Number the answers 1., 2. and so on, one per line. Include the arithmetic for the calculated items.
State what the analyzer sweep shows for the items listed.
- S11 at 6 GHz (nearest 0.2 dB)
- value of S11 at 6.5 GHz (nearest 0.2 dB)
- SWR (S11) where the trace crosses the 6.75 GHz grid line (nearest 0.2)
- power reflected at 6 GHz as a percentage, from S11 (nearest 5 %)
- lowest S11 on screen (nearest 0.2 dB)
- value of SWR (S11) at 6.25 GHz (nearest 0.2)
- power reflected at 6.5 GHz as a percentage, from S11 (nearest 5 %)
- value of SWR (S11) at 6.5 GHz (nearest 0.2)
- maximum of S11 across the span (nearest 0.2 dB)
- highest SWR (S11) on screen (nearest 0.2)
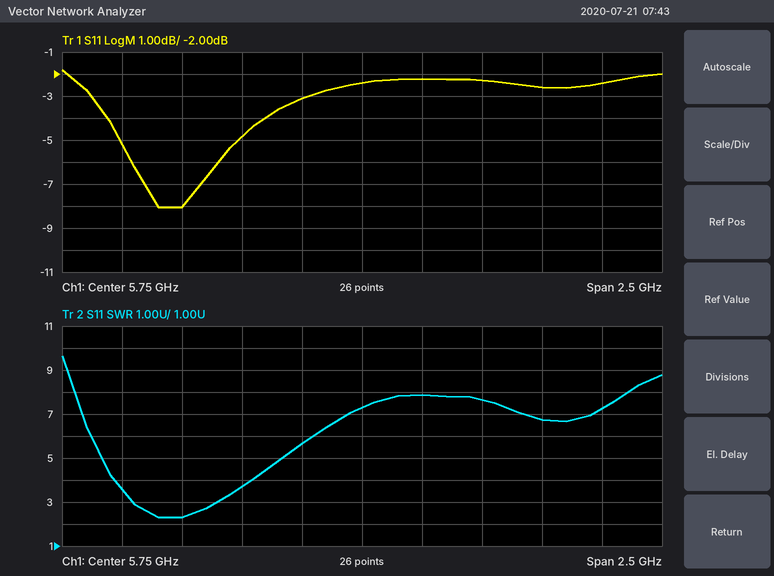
1. -2.2 dB
2. -2.6 dB
3. 7.2
4. 10^(-2.2/10) ≈ 60 %
5. -8.0 dB
6. 7.6
7. 10^(-2.6/10) ≈ 55 %
8. 6.8
9. -1.8 dB
10. 9.6
